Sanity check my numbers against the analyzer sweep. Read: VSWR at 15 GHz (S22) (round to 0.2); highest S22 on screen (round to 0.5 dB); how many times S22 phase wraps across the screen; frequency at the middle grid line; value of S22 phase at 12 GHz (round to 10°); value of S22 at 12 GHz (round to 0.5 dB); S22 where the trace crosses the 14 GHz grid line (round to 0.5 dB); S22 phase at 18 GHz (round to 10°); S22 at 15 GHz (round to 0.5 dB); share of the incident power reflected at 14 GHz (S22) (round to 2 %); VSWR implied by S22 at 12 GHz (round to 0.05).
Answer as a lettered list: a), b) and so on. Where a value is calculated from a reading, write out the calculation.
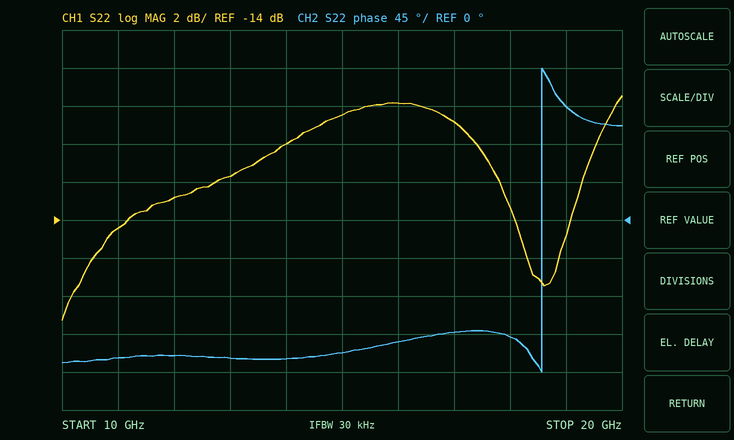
a) |Γ| = 10^(-8.5/20) = 0.3758; VSWR = (1 + 0.3758)/(1 − 0.3758) ≈ 2.2
b) -7.5 dB
c) 1
d) 15 GHz
e) -160°
f) -13.0 dB
g) -10.0 dB
h) -140°
i) -8.5 dB
j) 10^(-10/10) ≈ 10 %
k) |Γ| = 10^(-13/20) = 0.2239; VSWR = (1 + 0.2239)/(1 − 0.2239) ≈ 1.58, so 1.60 to the nearest 0.05
